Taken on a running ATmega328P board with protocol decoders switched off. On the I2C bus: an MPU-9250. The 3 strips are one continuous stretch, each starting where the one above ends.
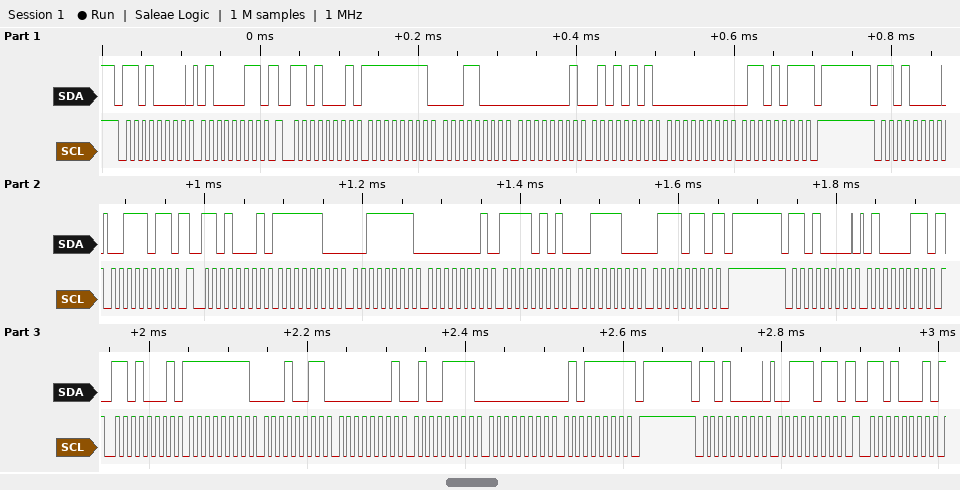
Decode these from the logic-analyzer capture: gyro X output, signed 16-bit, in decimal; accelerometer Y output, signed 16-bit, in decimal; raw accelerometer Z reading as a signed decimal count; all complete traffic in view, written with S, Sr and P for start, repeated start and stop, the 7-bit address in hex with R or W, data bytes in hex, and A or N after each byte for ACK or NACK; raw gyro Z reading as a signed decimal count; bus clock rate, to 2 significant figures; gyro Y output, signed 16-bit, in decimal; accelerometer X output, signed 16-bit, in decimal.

-232
501
15478
S 68W A 43 A Sr 68R A FF A 18 A 01 A 55 A 00 A 6B N P S 68W A 3B A Sr 68R A FC A 3F A 01 A F5 A 3C A 76 N P S 68W A 43 A Sr 68R A FF A 13 A 01 A 4F A 00 A 5F N P S 68W A 3B A Sr 68R A
107
100 kHz
341
-961
